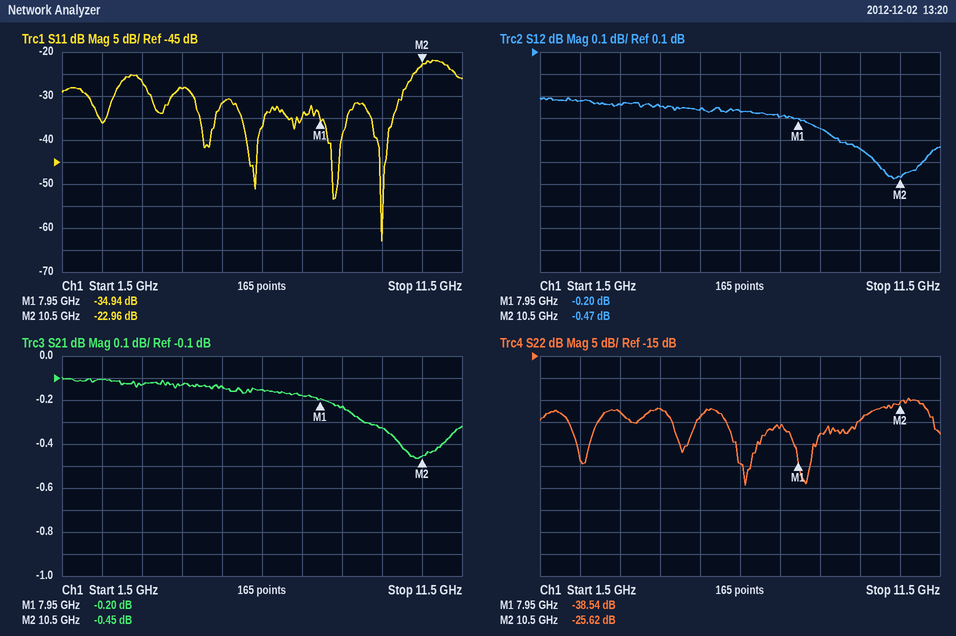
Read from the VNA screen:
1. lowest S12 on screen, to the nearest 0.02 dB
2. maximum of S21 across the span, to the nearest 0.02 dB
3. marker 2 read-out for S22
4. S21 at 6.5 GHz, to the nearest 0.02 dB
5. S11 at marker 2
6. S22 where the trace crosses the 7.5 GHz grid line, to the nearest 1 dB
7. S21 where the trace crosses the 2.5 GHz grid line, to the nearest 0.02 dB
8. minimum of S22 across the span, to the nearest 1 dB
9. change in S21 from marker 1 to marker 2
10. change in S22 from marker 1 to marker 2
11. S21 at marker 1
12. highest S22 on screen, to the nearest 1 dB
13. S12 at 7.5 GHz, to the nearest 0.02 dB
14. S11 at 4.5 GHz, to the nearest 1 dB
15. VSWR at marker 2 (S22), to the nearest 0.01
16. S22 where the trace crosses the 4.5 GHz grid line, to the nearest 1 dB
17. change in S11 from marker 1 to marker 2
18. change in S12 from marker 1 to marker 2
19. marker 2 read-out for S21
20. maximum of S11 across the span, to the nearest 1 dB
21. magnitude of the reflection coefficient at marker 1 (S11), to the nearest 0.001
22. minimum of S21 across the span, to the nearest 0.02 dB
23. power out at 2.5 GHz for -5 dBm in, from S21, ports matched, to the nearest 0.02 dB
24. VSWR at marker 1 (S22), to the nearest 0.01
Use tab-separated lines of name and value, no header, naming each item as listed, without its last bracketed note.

lowest S12 on screen, to the nearest 0.02 dB	-0.48 dB
maximum of S21 across the span, to the nearest 0.02 dB	-0.10 dB
marker 2 read-out for S22	-25.62 dB
S21 at 6.5 GHz, to the nearest 0.02 dB	-0.16 dB
S11 at marker 2	-22.96 dB
S22 where the trace crosses the 7.5 GHz grid line, to the nearest 1 dB	-31 dB
S21 where the trace crosses the 2.5 GHz grid line, to the nearest 0.02 dB	-0.10 dB
minimum of S22 across the span, to the nearest 1 dB	-44 dB
change in S21 from marker 1 to marker 2	-0.25 dB
change in S22 from marker 1 to marker 2	12.92 dB
S21 at marker 1	-0.20 dB
highest S22 on screen, to the nearest 1 dB	-25 dB
S12 at 7.5 GHz, to the nearest 0.02 dB	-0.20 dB
S11 at 4.5 GHz, to the nearest 1 dB	-28 dB
VSWR at marker 2 (S22), to the nearest 0.01	1.11
S22 where the trace crosses the 4.5 GHz grid line, to the nearest 1 dB	-27 dB
change in S11 from marker 1 to marker 2	11.98 dB
change in S12 from marker 1 to marker 2	-0.27 dB
marker 2 read-out for S21	-0.45 dB
maximum of S11 across the span, to the nearest 1 dB	-22 dB
magnitude of the reflection coefficient at marker 1 (S11), to the nearest 0.001	0.018
minimum of S21 across the span, to the nearest 0.02 dB	-0.46 dB
power out at 2.5 GHz for -5 dBm in, from S21, ports matched, to the nearest 0.02 dB	-5.10 dBm
VSWR at marker 1 (S22), to the nearest 0.01	1.02
